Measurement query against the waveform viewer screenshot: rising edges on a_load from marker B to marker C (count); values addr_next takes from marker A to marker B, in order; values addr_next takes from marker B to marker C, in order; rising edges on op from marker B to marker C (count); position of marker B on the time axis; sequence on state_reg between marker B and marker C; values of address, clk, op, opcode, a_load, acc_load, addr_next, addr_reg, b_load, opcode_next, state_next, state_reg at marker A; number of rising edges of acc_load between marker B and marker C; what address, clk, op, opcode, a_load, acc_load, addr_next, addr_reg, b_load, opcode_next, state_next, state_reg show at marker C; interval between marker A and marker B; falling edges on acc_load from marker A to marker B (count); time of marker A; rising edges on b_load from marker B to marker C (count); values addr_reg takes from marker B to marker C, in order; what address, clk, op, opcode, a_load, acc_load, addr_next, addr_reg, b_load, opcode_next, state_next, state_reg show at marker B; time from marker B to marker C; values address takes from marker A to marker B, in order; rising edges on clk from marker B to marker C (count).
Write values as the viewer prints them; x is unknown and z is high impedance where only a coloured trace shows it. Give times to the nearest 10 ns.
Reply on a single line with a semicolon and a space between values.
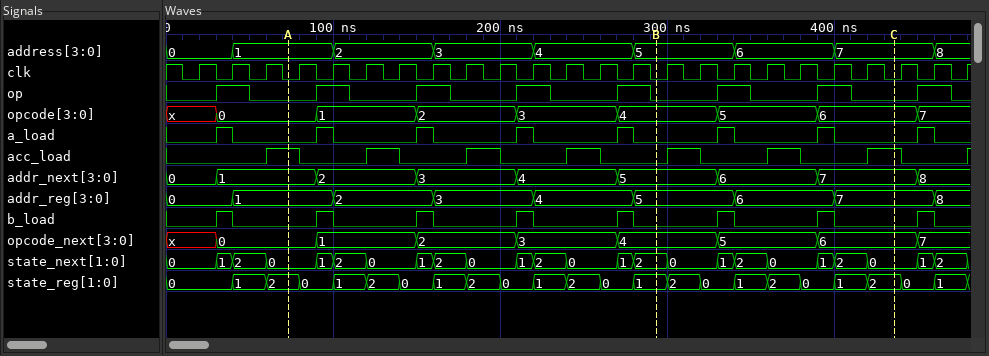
2; 1, 2, 3, 4, 5; 5, 6, 7; 2; 290 ns; 1, 2, 0, 1, 2, 0, 1, 2; address=1, clk=0, op=0, opcode=0, a_load=0, acc_load=1, addr_next=1, addr_reg=1, b_load=0, opcode_next=0, state_next=0, state_reg=2; 3; address=7, clk=0, op=0, opcode=6, a_load=0, acc_load=1, addr_next=7, addr_reg=7, b_load=0, opcode_next=6, state_next=0, state_reg=2; 220 ns; 4; 70 ns; 2; 5, 6, 7; address=5, clk=0, op=0, opcode=4, a_load=0, acc_load=0, addr_next=5, addr_reg=5, b_load=0, opcode_next=4, state_next=2, state_reg=1; 140 ns; 1, 2, 3, 4, 5; 7
